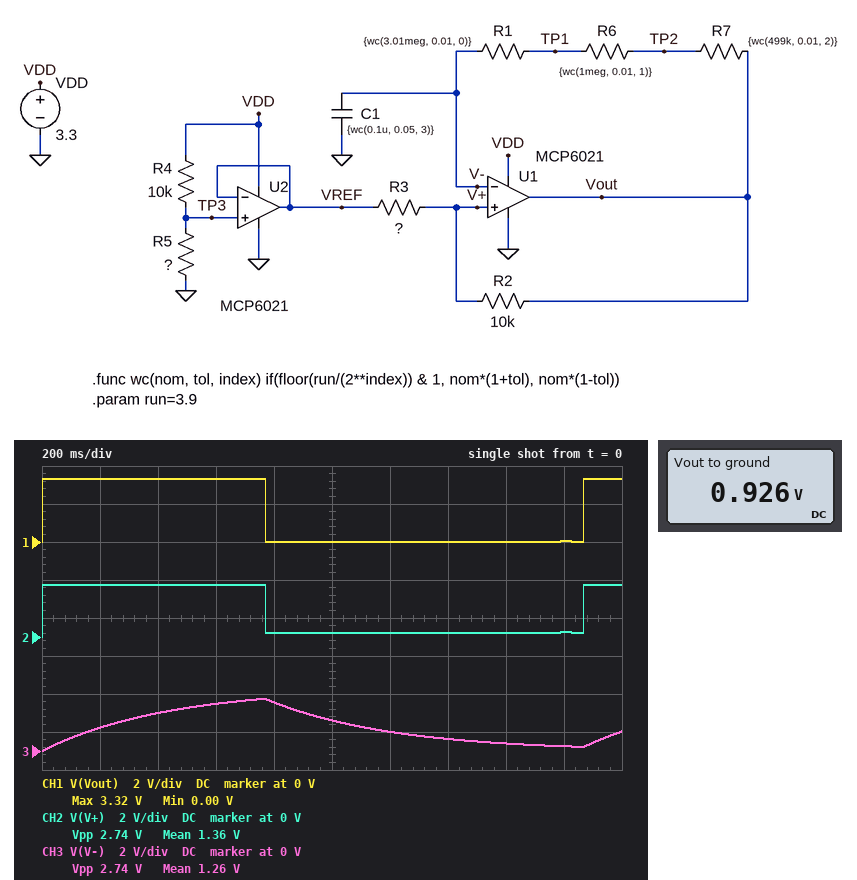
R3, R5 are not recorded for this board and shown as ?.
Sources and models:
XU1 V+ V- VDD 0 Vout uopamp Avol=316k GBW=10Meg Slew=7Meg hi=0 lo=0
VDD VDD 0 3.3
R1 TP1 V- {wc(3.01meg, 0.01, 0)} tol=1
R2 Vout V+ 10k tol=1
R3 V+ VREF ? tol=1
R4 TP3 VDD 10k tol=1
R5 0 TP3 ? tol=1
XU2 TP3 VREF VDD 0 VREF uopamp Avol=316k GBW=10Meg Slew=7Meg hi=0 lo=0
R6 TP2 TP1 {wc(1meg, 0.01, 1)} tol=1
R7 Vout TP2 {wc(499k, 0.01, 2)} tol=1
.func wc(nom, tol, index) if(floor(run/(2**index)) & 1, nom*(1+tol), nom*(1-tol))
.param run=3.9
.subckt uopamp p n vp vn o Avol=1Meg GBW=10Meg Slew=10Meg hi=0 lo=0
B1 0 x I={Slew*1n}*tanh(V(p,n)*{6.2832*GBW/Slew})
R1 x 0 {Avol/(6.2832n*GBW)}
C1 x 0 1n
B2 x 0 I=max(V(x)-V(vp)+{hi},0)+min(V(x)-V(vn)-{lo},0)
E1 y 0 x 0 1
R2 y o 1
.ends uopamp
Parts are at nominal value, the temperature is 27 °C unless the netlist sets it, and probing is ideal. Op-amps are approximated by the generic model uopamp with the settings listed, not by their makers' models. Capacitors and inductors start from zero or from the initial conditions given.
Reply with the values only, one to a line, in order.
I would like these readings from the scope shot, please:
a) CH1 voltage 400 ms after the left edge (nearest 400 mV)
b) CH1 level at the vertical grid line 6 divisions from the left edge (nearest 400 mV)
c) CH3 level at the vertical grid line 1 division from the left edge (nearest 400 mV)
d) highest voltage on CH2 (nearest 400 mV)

3.2 V
0 V
1.2 V
2.8 V
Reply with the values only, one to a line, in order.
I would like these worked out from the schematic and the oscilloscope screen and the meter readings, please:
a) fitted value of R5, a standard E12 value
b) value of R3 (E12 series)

3.9 kΩ
33 kΩ
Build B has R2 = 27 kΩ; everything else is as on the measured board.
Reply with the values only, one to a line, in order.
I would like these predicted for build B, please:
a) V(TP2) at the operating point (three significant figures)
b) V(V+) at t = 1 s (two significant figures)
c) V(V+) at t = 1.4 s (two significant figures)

926 mV
410 mV
2.2 V
